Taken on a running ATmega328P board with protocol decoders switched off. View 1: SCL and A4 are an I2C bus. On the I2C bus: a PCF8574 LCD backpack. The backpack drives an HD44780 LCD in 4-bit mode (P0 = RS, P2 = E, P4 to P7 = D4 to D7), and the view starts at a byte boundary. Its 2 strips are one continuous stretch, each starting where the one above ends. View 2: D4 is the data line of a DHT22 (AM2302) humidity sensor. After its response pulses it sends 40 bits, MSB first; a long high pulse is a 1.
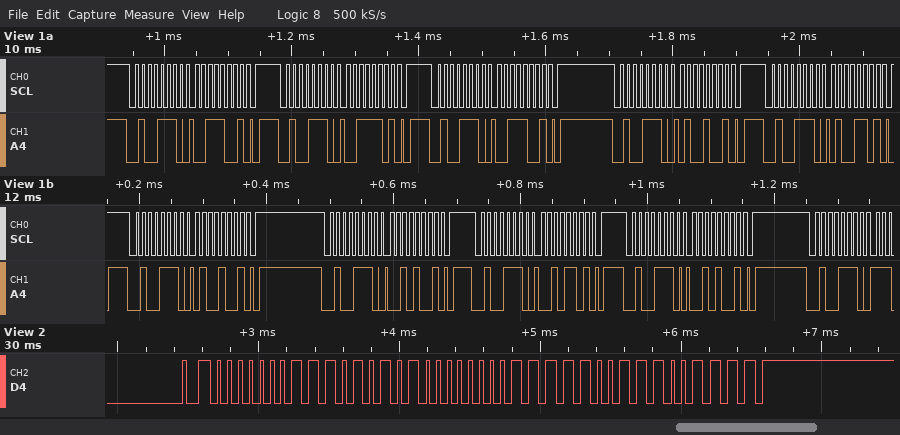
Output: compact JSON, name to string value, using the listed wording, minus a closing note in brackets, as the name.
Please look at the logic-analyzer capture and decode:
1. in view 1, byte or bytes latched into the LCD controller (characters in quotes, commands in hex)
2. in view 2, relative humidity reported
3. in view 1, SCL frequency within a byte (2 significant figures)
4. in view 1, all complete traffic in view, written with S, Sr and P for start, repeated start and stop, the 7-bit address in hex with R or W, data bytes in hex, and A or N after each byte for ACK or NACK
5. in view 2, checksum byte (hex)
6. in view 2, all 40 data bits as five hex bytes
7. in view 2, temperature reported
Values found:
{"in view 1, byte or bytes latched into the LCD controller": "'4'", "in view 2, relative humidity reported": "46.9 %", "in view 1, SCL frequency within a byte": "100 kHz", "in view 1, all complete traffic in view, written with S, Sr and P for start, repeated start and stop, the 7-bit address in hex with R or W, data bytes in hex, and A or N after each byte for ACK or NACK": "S 27W A 39 A P S 27W A 3D A P S 27W A 39 A P S 27W A 49 A P S 27W A 4D A P S 27W A 49 A P S 27W A 29 A P S 27W A 2D A P S 27W A 29 A P S 27W A", "in view 2, checksum byte": "0xCF", "in view 2, all 40 data bits as five hex bytes": "01 D5 00 F9 CF", "in view 2, temperature reported": "24.9 °C"}
